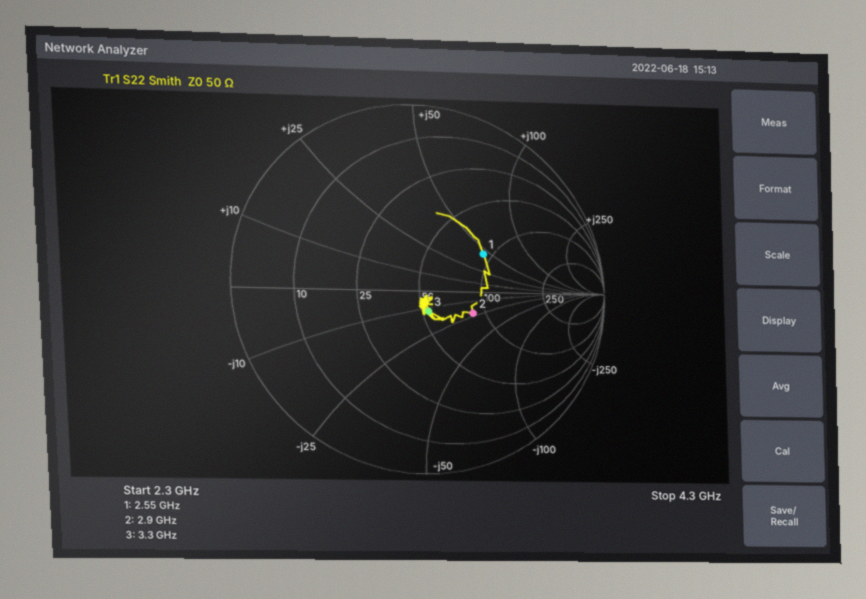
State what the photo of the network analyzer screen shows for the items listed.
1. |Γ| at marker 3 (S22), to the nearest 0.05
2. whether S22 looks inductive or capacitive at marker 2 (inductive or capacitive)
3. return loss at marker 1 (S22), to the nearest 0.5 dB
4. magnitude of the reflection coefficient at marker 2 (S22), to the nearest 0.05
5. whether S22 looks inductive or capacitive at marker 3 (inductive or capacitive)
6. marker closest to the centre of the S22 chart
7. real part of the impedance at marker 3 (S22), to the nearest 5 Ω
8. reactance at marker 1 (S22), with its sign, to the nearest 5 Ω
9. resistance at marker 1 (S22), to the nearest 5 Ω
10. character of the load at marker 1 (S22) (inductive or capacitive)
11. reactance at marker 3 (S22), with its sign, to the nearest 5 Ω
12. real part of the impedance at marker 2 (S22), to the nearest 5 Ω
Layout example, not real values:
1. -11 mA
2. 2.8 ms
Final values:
1. 0.10
2. capacitive
3. 8.0 dB
4. 0.30
5. capacitive
6. marker 3
7. 55 Ω
8. +45 Ω
9. 90 Ω
10. inductive
11. -10 Ω
12. 85 Ω
